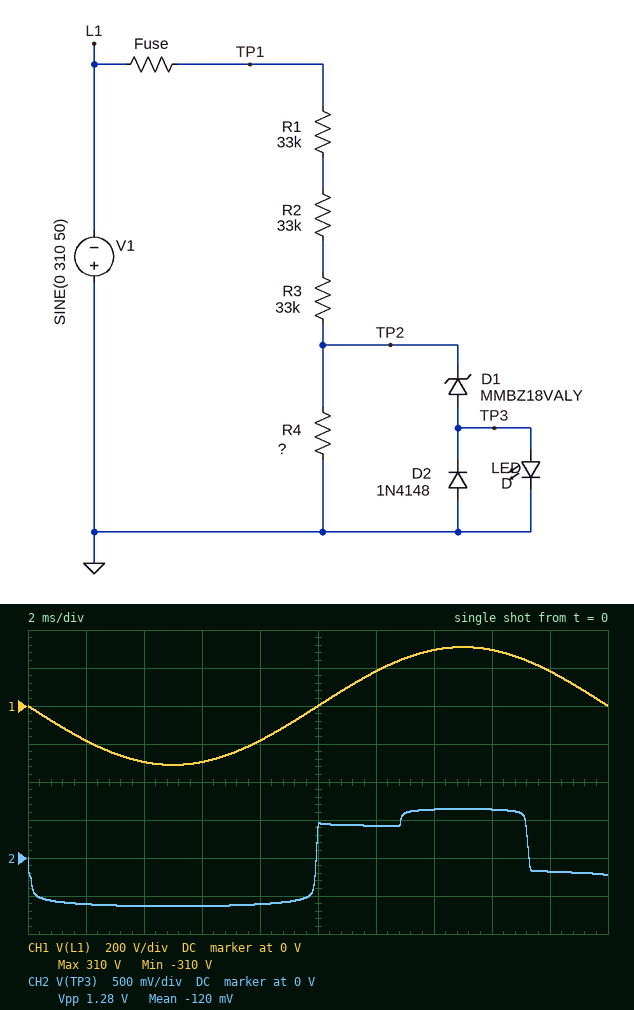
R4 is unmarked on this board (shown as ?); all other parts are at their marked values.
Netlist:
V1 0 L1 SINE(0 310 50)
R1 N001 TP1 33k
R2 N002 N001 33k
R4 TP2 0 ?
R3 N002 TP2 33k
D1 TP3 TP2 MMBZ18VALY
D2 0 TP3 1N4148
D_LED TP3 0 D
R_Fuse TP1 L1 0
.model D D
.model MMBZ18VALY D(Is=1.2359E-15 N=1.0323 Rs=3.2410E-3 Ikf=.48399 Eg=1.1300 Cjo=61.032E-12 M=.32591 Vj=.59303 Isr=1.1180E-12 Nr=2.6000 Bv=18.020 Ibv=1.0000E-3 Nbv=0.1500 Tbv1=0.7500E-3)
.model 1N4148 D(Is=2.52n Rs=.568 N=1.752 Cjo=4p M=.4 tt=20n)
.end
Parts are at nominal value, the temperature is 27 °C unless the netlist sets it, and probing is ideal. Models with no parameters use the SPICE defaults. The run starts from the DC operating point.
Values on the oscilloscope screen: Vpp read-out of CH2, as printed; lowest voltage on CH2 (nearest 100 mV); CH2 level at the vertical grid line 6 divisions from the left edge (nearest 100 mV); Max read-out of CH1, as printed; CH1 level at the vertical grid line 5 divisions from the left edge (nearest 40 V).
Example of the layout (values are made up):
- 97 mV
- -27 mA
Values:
- 1.28 V
- -600 mV
- 400 mV
- 310 V
- 0 V
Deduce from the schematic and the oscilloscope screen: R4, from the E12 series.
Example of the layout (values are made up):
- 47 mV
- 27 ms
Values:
- 8.2 kΩ
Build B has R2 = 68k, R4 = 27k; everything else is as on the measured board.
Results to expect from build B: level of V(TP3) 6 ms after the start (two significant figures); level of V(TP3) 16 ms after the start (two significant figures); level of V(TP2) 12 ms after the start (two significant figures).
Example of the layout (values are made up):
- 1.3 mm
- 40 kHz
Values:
- -620 mV
- 660 mV
- 19 V
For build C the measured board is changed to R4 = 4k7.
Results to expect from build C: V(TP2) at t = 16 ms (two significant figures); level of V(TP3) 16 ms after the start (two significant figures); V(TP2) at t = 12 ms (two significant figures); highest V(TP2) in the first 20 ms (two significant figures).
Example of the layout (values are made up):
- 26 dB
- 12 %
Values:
- 13 V
- -110 mV
- 8.3 V
- 14 V
